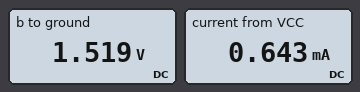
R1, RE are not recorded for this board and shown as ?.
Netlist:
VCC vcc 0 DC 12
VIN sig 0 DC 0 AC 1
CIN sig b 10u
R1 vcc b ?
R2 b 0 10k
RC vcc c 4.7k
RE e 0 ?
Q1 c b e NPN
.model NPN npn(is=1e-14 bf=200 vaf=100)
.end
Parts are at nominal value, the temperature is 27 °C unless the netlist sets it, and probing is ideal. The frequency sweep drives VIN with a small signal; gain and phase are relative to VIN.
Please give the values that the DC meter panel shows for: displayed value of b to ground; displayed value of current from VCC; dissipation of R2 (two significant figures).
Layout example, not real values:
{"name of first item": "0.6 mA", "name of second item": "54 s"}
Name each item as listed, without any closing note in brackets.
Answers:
{"displayed value of b to ground": "1.519 V", "displayed value of current from VCC": "0.643 mA", "dissipation of R2": "230 µW"}
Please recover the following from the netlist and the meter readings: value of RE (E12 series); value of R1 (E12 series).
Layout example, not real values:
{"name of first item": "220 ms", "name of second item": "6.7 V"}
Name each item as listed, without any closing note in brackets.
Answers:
{"value of RE": "1.8 kΩ", "value of R1": "68 kΩ"}
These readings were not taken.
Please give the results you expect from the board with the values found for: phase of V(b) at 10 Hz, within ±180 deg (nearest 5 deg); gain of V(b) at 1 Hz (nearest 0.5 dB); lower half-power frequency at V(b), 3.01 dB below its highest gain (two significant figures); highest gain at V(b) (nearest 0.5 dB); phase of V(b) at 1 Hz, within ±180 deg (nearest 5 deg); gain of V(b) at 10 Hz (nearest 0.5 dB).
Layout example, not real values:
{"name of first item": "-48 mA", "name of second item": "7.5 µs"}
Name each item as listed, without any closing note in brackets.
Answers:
{"phase of V(b) at 10 Hz, within ±180 deg": "10 deg", "gain of V(b) at 1 Hz": "-6.5 dB", "lower half-power frequency at V(b), 3.01 dB below its highest gain": "1.9 Hz", "highest gain at V(b)": "0 dB", "phase of V(b) at 1 Hz, within ±180 deg": "60 deg", "gain of V(b) at 10 Hz": "0 dB"}
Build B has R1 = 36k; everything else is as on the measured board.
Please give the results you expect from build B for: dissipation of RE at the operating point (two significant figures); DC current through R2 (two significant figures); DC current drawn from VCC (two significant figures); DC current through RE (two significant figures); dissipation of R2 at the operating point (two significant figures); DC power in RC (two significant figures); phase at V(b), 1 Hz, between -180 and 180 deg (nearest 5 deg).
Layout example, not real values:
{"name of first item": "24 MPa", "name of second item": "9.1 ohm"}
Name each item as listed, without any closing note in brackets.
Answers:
{"dissipation of RE at the operating point": "2.0 mW", "DC current through R2": "260 µA", "DC current drawn from VCC": "1.3 mA", "DC current through RE": "1.1 mA", "dissipation of R2 at the operating point": "660 µW", "DC power in RC": "5.3 mW", "phase at V(b), 1 Hz, between -180 and 180 deg": "65 deg"}
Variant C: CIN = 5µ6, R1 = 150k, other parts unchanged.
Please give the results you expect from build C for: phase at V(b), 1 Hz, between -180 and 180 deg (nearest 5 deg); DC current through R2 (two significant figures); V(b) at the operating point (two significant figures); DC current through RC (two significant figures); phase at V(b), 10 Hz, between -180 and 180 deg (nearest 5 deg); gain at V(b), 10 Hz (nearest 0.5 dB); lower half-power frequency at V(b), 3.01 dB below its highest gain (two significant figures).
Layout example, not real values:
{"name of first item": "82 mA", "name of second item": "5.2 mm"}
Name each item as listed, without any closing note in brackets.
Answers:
{"phase at V(b), 1 Hz, between -180 and 180 deg": "70 deg", "DC current through R2": "75 µA", "V(b) at the operating point": "750 mV", "DC current through RC": "87 µA", "phase at V(b), 10 Hz, between -180 and 180 deg": "15 deg", "gain at V(b), 10 Hz": "-0.5 dB", "lower half-power frequency at V(b), 3.01 dB below its highest gain": "3.1 Hz"}
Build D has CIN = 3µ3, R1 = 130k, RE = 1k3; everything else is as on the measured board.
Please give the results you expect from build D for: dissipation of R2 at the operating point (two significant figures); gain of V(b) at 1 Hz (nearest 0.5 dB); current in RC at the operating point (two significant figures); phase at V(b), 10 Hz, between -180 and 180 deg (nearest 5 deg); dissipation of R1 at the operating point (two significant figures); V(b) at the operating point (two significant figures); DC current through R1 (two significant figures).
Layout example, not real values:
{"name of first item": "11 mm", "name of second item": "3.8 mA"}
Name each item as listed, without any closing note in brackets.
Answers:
{"dissipation of R2 at the operating point": "72 µW", "gain of V(b) at 1 Hz": "-14.5 dB", "current in RC at the operating point": "180 µA", "phase at V(b), 10 Hz, between -180 and 180 deg": "30 deg", "dissipation of R1 at the operating point": "960 µW", "V(b) at the operating point": "850 mV", "DC current through R1": "86 µA"}
